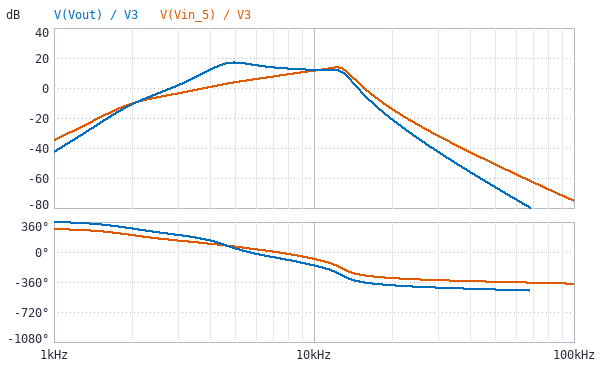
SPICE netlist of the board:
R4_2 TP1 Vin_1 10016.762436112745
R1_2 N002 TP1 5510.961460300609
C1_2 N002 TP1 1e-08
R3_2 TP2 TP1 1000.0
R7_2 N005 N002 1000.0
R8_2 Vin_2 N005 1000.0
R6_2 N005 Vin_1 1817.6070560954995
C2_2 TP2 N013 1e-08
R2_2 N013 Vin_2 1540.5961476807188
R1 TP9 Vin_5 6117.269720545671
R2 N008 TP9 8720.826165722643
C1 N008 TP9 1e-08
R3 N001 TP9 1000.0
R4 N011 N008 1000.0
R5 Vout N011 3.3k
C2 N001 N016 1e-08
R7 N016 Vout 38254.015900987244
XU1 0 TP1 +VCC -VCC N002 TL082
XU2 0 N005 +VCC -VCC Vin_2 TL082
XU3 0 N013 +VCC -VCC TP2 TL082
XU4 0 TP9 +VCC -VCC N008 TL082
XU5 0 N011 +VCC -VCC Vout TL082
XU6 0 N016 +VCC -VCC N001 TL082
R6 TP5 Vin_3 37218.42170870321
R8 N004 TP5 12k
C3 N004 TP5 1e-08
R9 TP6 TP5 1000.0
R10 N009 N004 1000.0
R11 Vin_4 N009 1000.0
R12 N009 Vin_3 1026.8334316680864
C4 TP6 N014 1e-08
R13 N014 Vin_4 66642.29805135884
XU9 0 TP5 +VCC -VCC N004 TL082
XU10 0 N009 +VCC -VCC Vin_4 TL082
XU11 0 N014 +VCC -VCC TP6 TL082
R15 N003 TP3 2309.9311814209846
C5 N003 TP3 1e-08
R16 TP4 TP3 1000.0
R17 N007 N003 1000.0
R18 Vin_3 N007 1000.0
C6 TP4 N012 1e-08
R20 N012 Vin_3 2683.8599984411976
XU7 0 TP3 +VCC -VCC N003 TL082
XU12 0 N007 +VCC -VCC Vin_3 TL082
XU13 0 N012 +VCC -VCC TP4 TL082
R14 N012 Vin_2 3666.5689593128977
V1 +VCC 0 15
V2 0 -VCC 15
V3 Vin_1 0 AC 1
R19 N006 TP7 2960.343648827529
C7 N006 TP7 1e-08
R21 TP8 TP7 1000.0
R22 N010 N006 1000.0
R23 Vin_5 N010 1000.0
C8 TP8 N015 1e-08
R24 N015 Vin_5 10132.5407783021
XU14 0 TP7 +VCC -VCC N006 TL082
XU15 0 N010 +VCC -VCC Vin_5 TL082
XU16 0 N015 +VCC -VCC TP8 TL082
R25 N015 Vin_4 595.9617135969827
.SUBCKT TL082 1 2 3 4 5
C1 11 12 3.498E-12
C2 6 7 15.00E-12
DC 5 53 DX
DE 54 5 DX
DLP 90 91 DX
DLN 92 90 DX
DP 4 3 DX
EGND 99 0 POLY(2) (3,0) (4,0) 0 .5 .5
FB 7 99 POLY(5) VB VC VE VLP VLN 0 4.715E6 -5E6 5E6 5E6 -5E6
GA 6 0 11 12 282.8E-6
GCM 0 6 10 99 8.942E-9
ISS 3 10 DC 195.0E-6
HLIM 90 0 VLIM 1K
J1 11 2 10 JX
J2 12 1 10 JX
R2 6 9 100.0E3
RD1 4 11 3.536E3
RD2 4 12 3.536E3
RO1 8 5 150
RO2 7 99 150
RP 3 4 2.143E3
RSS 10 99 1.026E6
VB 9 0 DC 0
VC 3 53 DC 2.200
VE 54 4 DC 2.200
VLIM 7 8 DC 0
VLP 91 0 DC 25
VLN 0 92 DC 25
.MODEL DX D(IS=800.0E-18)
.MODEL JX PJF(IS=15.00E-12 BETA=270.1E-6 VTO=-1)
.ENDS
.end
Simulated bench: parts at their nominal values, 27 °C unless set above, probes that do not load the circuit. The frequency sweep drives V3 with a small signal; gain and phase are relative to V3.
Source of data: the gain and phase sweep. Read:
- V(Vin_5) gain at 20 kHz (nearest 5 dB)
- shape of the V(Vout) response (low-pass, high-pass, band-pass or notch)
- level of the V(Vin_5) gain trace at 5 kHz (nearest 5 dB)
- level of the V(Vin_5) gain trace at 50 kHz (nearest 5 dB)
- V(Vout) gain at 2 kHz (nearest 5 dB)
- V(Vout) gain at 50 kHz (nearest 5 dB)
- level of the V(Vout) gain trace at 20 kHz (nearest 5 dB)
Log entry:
-15 dB
band-pass
5 dB
-50 dB
-10 dB
-65 dB
-20 dB
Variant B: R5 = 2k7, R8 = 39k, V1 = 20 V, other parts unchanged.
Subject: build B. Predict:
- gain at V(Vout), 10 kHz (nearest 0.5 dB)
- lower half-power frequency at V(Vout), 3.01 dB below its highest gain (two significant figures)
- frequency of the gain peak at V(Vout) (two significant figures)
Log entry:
10.0 dB
3.8 kHz
4.5 kHz
